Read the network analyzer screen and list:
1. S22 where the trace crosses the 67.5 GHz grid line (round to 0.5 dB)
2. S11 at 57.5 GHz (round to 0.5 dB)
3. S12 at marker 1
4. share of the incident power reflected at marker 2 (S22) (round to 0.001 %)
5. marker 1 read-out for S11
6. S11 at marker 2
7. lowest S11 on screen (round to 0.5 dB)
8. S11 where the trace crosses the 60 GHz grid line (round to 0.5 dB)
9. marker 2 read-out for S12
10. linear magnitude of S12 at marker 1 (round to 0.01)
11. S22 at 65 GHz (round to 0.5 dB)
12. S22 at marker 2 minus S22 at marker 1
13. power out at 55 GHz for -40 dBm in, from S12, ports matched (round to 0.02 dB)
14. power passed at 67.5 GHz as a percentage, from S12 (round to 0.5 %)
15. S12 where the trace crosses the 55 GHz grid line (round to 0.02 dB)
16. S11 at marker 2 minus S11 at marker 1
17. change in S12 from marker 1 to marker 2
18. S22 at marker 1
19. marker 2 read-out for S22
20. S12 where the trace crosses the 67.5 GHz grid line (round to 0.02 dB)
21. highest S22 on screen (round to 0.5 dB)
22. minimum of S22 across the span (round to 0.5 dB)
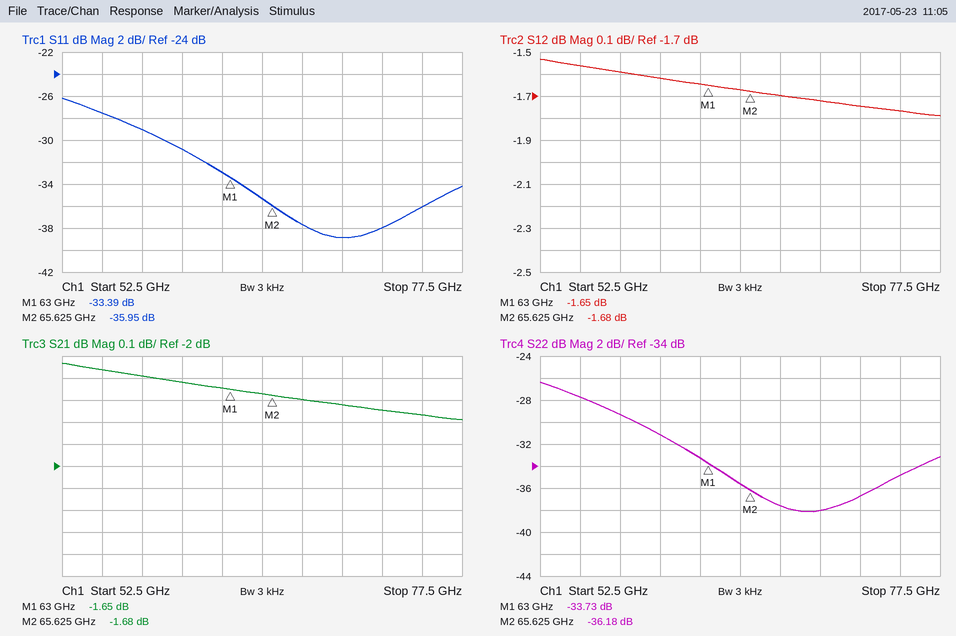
-37.5 dB
-29.0 dB
-1.65 dB
0.024 %
-33.39 dB
-35.95 dB
-39.0 dB
-31.0 dB
-1.68 dB
0.83
-35.5 dB
-2.45 dB
-41.56 dBm
67.5 %
-1.56 dB
-2.56 dB
-0.03 dB
-33.73 dB
-36.18 dB
-1.70 dB
-26.5 dB
-38.0 dB
